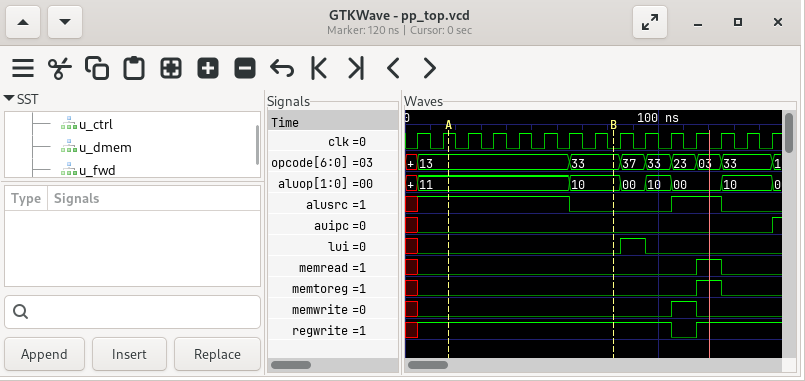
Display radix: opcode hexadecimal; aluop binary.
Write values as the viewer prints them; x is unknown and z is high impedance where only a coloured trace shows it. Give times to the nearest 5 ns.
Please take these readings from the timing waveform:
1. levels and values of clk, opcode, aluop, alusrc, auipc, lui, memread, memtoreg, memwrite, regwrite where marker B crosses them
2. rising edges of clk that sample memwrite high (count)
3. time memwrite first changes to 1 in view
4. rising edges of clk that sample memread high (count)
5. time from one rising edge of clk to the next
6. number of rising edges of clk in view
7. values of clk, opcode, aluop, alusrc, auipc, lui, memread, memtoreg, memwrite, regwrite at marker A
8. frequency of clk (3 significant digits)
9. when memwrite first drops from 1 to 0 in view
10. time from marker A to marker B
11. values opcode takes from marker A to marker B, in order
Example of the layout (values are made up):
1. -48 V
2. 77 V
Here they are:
1. clk=0, opcode=33, aluop=10, alusrc=0, auipc=0, lui=0, memread=0, memtoreg=0, memwrite=0, regwrite=1
2. 1
3. 105 ns
4. 1
5. 10 ns
6. 15
7. clk=1, opcode=13, aluop=11, alusrc=1, auipc=0, lui=0, memread=0, memtoreg=0, memwrite=0, regwrite=1
8. 100 MHz
9. 115 ns
10. 65 ns
11. 13, 33
